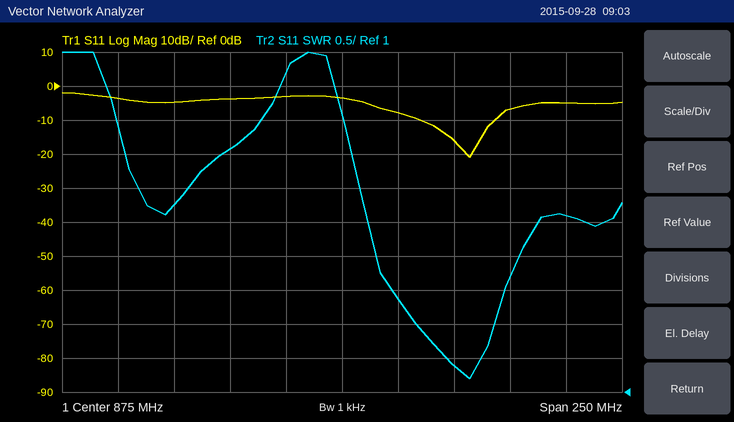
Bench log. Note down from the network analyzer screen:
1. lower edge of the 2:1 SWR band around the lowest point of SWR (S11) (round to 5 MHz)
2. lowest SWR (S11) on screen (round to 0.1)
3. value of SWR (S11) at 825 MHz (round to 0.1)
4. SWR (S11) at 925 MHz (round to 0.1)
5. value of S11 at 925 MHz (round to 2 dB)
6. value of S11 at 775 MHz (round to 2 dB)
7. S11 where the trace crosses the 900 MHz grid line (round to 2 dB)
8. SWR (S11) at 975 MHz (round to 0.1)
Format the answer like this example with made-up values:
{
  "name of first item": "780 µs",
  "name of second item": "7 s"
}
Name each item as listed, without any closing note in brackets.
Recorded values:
{
  "lower edge of the 2:1 SWR band around the lowest point of SWR (S11)": "910 MHz",
  "lowest SWR (S11) on screen": "1.2",
  "value of SWR (S11) at 825 MHz": "4.6",
  "SWR (S11) at 925 MHz": "1.4",
  "value of S11 at 925 MHz": "-16 dB",
  "value of S11 at 775 MHz": "-4 dB",
  "S11 where the trace crosses the 900 MHz grid line": "-8 dB",
  "SWR (S11) at 975 MHz": "3.6"
}
